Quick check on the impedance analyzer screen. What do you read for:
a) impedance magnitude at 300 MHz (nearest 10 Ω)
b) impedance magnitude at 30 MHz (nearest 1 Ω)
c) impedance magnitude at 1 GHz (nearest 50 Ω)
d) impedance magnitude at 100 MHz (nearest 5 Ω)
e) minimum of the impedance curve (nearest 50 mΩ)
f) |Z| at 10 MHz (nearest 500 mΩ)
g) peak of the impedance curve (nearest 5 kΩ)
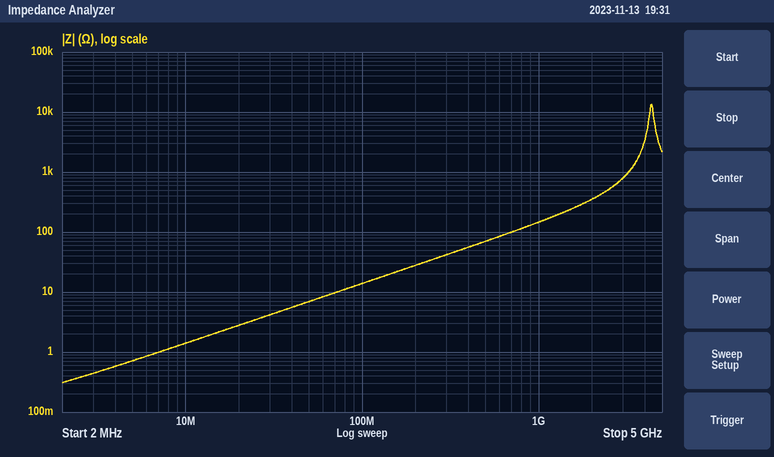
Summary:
40 Ω
4 Ω
150 Ω
15 Ω
300 mΩ
1.5 Ω
15 kΩ
